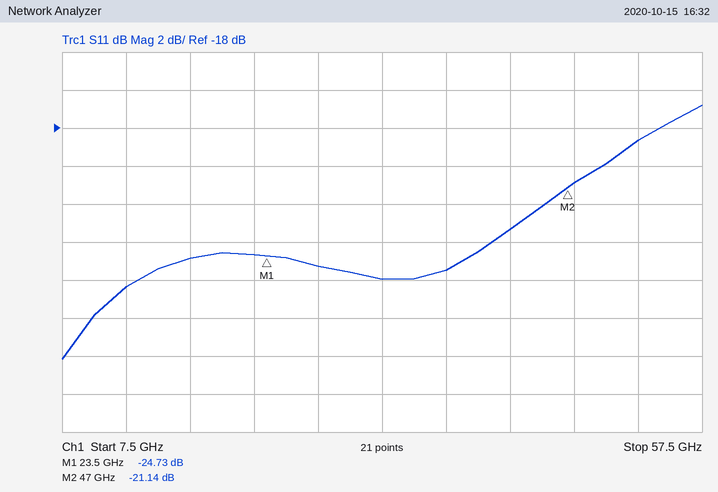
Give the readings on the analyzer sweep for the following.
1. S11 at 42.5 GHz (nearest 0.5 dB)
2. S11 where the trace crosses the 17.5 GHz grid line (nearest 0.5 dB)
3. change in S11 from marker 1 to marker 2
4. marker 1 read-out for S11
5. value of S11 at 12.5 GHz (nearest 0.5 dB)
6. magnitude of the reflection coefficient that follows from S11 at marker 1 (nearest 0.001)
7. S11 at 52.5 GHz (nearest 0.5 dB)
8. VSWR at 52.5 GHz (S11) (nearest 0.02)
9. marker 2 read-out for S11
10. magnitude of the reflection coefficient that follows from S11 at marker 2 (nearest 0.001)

-23.5 dB
-25.0 dB
3.59 dB
-24.73 dB
-26.5 dB
0.058
-18.5 dB
1.26
-21.14 dB
0.088
